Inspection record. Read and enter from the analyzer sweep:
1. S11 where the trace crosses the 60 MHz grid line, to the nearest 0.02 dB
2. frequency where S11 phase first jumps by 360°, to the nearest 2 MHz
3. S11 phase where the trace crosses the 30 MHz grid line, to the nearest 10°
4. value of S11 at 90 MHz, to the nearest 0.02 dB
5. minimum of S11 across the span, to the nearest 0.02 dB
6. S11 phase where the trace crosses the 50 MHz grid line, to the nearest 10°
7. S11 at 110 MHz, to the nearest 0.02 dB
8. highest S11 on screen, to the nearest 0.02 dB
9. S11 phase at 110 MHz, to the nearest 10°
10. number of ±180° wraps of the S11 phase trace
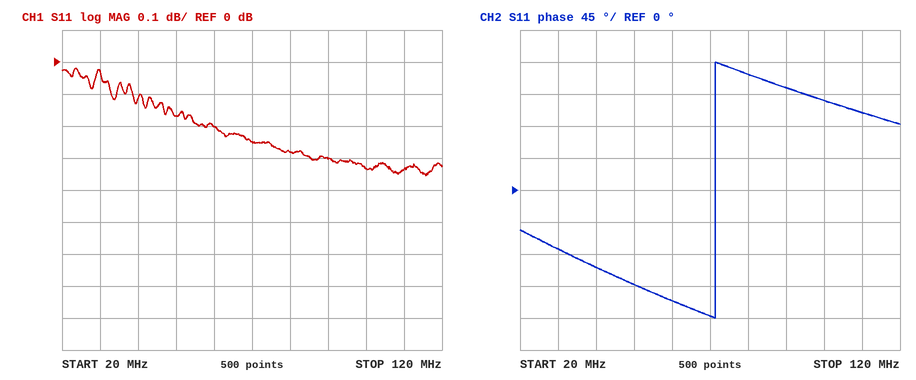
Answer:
-0.20 dB
72 MHz
-80°
-0.30 dB
-0.36 dB
-130°
-0.34 dB
-0.02 dB
110°
1
